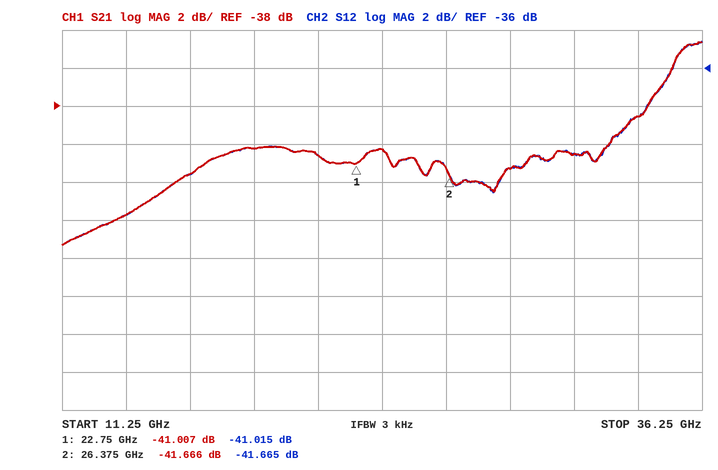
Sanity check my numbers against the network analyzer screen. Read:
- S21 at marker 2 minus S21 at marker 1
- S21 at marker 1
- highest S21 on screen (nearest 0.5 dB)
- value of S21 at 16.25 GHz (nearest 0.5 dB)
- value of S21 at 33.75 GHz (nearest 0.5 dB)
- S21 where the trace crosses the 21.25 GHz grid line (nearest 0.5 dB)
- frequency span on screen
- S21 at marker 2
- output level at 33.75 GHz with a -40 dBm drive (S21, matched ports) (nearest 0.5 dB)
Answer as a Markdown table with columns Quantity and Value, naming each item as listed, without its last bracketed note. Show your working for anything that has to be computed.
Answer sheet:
| Quantity | Value |
|---|---|
| S21 at marker 2 minus S21 at marker 1 | -41.666 − (-41.007) = -0.659 dB |
| S21 at marker 1 | -41.007 dB |
| highest S21 on screen | -34.5 dB |
| value of S21 at 16.25 GHz | -41.5 dB |
| value of S21 at 33.75 GHz | -38.5 dB |
| S21 where the trace crosses the 21.25 GHz grid line | -40.5 dB |
| frequency span on screen | 25 GHz |
| S21 at marker 2 | -41.666 dB |
| output level at 33.75 GHz with a -40 dBm drive (S21, matched ports) | -40 dBm + (-38.5 dB) = -78.5 dBm |
